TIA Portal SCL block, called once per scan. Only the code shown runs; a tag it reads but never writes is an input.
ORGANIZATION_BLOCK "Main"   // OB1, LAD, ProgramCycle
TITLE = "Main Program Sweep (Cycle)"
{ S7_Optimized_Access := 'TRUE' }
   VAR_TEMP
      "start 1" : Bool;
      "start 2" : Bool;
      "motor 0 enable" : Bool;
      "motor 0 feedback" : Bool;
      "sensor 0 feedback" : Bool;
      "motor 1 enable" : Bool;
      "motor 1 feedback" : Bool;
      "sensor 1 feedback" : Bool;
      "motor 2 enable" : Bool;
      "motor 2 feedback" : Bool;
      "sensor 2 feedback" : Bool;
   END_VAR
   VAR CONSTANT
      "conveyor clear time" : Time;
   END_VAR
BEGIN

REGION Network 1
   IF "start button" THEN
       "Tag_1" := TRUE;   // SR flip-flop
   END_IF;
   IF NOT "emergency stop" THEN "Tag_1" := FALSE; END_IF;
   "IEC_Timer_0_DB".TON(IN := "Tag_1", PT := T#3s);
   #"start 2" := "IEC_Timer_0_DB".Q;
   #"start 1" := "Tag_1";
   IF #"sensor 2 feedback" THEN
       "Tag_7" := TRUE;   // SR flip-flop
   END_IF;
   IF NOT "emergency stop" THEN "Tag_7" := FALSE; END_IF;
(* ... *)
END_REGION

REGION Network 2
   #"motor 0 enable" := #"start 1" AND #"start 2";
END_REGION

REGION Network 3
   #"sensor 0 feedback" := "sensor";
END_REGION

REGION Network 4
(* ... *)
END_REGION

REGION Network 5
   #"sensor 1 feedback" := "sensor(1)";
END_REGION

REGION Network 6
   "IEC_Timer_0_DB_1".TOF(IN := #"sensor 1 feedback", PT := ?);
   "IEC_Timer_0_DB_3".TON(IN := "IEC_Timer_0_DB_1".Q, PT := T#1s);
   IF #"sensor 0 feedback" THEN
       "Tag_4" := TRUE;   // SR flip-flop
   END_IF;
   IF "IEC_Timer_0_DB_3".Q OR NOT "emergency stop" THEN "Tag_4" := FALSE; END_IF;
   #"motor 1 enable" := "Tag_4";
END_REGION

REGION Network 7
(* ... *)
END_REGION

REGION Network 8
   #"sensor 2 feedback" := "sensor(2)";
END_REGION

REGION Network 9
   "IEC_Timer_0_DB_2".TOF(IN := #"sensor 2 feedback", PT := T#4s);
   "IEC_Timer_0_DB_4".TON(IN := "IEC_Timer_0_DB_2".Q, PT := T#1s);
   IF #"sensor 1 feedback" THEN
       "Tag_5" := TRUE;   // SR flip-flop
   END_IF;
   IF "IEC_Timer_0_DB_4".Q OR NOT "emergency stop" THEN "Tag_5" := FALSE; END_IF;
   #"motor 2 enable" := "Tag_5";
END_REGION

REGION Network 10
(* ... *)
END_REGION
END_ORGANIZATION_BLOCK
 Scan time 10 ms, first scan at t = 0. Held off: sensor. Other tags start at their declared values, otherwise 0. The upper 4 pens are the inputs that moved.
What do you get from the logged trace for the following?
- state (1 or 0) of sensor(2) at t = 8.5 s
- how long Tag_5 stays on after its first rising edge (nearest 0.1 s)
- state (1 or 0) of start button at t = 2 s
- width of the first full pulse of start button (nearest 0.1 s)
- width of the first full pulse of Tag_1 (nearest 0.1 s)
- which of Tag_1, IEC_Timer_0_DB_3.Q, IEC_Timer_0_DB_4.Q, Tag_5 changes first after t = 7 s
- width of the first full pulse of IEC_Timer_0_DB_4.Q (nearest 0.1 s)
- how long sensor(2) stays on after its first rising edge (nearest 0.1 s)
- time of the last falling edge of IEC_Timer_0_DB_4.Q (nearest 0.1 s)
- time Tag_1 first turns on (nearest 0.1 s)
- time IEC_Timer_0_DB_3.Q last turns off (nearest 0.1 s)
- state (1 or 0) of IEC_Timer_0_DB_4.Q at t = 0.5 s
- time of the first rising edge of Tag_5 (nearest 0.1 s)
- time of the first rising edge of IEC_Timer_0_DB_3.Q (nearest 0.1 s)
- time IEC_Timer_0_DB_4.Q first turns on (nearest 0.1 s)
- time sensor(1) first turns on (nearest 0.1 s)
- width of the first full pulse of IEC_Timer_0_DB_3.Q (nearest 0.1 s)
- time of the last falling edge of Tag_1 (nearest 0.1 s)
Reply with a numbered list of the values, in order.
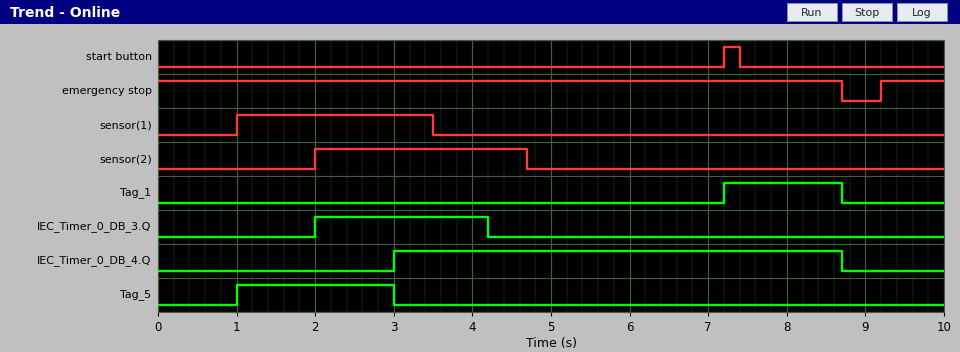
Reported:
1. 0
2. 2.0 s
3. 0
4. 0.2 s
5. 1.5 s
6. Tag_1
7. 5.7 s
8. 2.7 s
9. 8.7 s
10. 7.2 s
11. 4.2 s
12. 0
13. 1.0 s
14. 2.0 s
15. 3.0 s
16. 1.0 s
17. 2.2 s
18. 8.7 s
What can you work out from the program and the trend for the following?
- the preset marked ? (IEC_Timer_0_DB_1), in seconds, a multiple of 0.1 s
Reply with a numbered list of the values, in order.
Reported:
1. 0.7 s
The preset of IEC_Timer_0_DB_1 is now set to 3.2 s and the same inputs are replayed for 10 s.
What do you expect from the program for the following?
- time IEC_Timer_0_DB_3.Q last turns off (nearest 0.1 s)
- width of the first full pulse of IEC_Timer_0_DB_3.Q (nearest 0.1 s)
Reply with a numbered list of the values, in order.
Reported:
1. 6.7 s
2. 4.7 s
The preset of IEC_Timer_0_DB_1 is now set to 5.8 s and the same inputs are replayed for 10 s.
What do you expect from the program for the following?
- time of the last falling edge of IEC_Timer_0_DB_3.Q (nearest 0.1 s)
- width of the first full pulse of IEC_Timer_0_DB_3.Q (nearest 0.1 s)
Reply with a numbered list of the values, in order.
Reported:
1. 9.3 s
2. 7.3 s
